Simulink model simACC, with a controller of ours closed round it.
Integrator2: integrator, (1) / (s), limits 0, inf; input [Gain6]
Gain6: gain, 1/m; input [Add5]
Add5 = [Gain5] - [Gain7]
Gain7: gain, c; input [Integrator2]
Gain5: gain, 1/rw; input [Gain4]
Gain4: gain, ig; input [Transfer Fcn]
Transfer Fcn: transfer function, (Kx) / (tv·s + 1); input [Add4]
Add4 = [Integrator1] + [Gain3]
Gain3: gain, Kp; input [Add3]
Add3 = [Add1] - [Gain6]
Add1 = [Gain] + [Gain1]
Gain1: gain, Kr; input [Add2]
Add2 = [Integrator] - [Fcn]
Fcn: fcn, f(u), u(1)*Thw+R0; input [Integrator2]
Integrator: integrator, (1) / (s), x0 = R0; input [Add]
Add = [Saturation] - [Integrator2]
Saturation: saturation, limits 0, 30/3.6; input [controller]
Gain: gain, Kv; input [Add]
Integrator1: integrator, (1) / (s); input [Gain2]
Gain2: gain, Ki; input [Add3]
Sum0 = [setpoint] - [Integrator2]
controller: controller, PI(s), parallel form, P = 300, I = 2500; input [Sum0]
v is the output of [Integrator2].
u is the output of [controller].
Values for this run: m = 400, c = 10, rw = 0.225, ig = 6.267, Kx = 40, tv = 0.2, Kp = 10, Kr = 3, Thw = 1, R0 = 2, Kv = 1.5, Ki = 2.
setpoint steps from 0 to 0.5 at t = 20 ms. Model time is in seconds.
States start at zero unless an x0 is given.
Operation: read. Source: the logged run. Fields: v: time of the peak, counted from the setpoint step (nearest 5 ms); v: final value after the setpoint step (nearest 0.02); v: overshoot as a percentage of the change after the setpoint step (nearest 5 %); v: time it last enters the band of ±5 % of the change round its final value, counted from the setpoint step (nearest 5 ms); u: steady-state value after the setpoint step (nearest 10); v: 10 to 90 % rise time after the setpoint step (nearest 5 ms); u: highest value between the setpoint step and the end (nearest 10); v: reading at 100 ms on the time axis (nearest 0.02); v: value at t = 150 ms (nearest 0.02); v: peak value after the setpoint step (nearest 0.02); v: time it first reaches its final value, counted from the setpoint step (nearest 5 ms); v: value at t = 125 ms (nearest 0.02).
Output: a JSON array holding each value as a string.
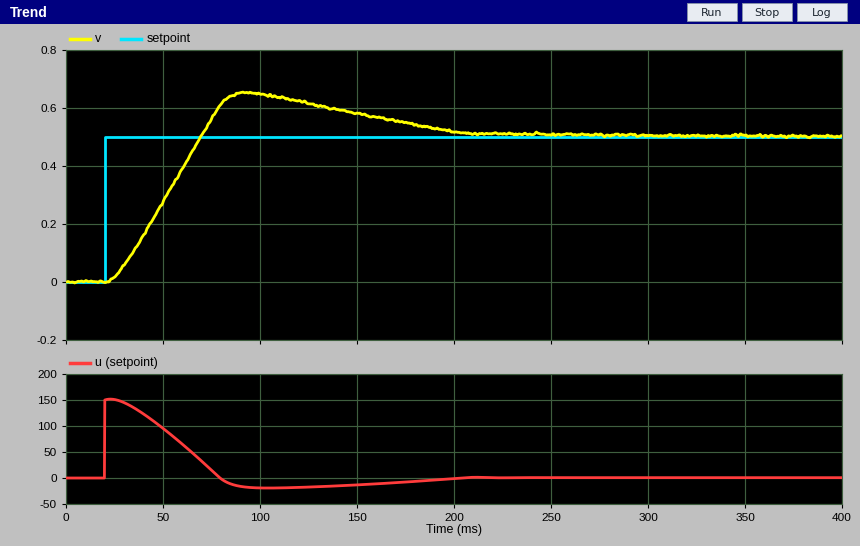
["75 ms", "0.50", "30 %", "175 ms", "0", "35 ms", "150", "0.64", "0.58", "0.66", "50 ms", "0.62"]
